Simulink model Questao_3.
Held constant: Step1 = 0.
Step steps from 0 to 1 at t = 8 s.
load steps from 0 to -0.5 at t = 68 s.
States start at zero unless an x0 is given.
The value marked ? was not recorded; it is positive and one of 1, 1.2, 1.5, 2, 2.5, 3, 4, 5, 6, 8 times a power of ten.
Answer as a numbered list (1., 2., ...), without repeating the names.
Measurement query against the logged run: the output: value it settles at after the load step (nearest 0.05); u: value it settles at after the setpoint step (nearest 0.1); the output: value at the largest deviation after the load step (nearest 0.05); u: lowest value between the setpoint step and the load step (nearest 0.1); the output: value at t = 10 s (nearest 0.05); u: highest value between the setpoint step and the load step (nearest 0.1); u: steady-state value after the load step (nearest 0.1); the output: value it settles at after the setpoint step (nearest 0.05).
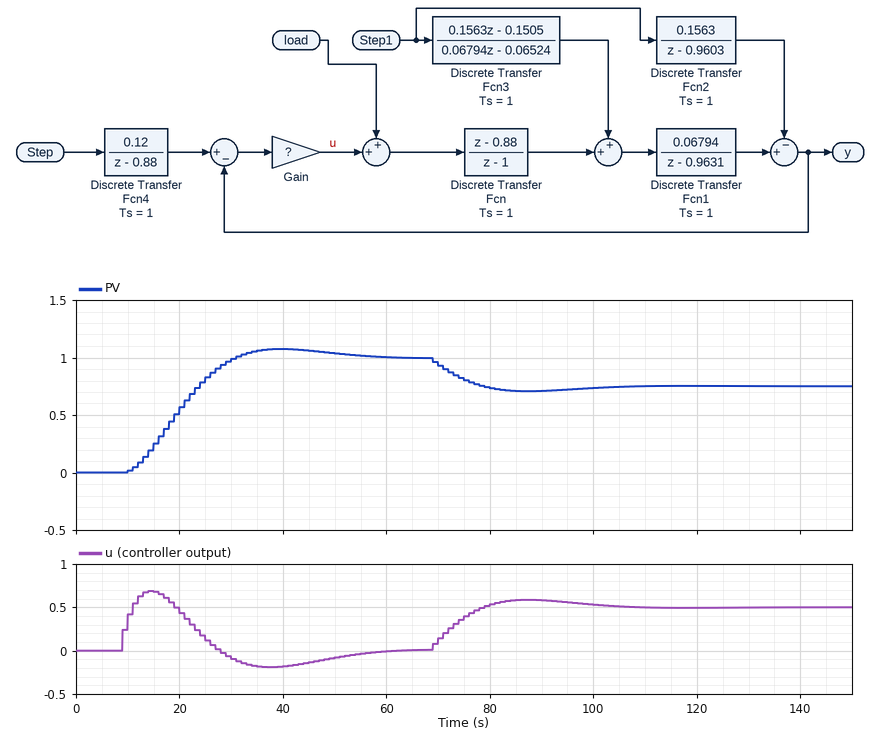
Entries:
1. 0.75
2. 0.0
3. 0.70
4. -0.2
5. 0.00
6. 0.7
7. 0.5
8. 1.00
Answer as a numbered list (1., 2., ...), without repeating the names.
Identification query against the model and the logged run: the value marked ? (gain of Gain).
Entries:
1. 2
